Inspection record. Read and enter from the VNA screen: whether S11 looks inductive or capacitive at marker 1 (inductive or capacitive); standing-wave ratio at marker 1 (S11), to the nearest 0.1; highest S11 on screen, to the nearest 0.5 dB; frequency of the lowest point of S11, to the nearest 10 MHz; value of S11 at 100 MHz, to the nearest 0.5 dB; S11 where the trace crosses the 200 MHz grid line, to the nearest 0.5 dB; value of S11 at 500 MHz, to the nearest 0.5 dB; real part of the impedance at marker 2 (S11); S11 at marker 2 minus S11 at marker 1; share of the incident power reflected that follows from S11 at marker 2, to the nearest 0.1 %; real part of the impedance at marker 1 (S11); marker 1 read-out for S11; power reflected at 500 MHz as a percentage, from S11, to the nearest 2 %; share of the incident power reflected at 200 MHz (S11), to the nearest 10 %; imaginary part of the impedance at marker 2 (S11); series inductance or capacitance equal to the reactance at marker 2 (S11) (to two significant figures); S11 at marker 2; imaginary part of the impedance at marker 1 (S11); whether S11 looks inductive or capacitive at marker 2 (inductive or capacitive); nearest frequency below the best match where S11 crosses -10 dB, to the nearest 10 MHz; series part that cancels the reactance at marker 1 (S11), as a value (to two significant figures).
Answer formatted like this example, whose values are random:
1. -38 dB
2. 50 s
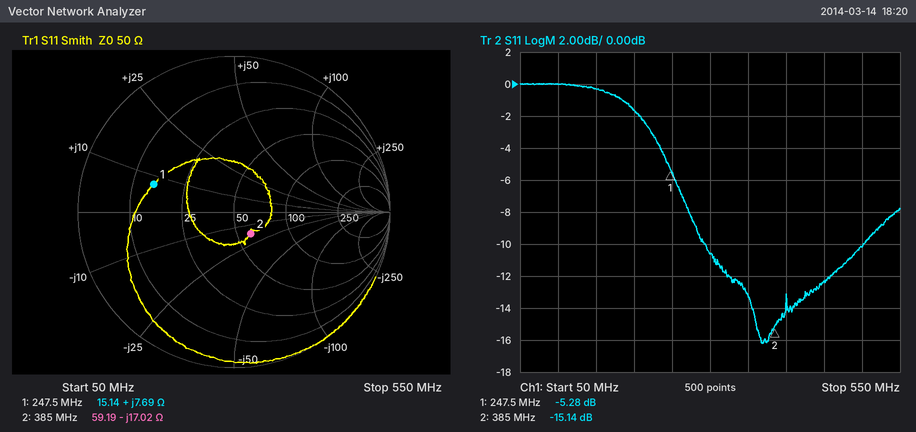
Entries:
1. inductive
2. 3.4
3. 0.0 dB
4. 370 MHz
5. 0.0 dB
6. -1.5 dB
7. -10.0 dB
8. 59.19 Ω
9. -9.86 dB
10. 3.1 %
11. 15.14 Ω
12. -5.28 dB
13. 10 %
14. 70 %
15. -17.02 Ω
16. 24 pF
17. -15.14 dB
18. +7.69 Ω
19. capacitive
20. 290 MHz
21. 84 pF
